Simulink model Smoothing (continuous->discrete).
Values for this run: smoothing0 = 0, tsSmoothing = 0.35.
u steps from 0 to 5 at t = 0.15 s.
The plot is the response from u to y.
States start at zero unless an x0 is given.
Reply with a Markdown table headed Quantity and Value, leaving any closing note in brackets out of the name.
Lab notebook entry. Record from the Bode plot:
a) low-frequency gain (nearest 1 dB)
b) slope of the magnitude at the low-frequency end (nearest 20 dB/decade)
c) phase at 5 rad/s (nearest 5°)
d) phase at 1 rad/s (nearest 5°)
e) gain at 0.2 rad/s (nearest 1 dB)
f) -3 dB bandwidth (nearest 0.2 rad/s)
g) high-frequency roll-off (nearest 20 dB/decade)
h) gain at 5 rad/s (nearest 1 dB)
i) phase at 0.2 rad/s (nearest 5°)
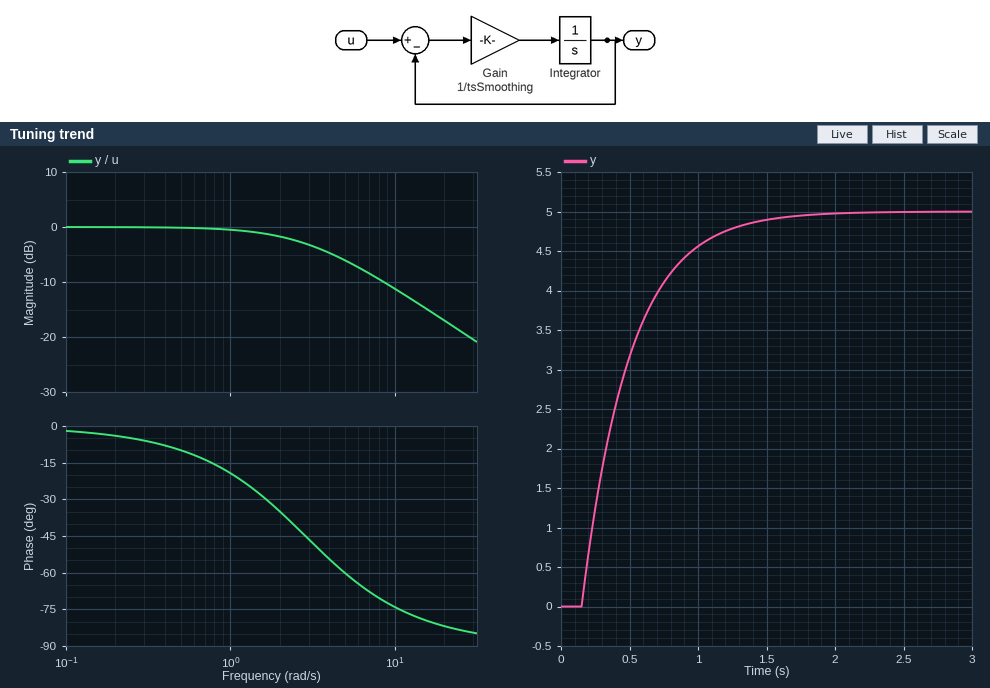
| Quantity | Value |
|---|---|
| low-frequency gain | 0 dB |
| slope of the magnitude at the low-frequency end | 0 dB/decade |
| phase at 5 rad/s | -60° |
| phase at 1 rad/s | -20° |
| gain at 0.2 rad/s | 0 dB |
| -3 dB bandwidth | 2.8 rad/s |
| high-frequency roll-off | -20 dB/decade |
| gain at 5 rad/s | -6 dB |
| phase at 0.2 rad/s | -5° |
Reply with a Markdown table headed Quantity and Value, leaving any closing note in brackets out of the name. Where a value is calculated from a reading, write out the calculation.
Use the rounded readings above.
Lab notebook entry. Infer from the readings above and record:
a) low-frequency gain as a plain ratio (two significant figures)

| Quantity | Value |
|---|---|
| low-frequency gain as a plain ratio | 10^(0 / 20) = 1.0 |
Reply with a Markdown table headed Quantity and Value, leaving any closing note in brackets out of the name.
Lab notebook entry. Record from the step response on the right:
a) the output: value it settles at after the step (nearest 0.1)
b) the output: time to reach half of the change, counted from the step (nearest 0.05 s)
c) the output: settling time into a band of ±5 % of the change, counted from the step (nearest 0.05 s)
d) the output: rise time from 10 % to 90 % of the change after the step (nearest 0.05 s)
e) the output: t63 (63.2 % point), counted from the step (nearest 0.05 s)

| Quantity | Value |
|---|---|
| the output: value it settles at after the step | 5.0 |
| the output: time to reach half of the change, counted from the step | 0.25 s |
| the output: settling time into a band of ±5 % of the change, counted from the step | 1.05 s |
| the output: rise time from 10 % to 90 % of the change after the step | 0.75 s |
| the output: t63 (63.2 % point), counted from the step | 0.35 s |
